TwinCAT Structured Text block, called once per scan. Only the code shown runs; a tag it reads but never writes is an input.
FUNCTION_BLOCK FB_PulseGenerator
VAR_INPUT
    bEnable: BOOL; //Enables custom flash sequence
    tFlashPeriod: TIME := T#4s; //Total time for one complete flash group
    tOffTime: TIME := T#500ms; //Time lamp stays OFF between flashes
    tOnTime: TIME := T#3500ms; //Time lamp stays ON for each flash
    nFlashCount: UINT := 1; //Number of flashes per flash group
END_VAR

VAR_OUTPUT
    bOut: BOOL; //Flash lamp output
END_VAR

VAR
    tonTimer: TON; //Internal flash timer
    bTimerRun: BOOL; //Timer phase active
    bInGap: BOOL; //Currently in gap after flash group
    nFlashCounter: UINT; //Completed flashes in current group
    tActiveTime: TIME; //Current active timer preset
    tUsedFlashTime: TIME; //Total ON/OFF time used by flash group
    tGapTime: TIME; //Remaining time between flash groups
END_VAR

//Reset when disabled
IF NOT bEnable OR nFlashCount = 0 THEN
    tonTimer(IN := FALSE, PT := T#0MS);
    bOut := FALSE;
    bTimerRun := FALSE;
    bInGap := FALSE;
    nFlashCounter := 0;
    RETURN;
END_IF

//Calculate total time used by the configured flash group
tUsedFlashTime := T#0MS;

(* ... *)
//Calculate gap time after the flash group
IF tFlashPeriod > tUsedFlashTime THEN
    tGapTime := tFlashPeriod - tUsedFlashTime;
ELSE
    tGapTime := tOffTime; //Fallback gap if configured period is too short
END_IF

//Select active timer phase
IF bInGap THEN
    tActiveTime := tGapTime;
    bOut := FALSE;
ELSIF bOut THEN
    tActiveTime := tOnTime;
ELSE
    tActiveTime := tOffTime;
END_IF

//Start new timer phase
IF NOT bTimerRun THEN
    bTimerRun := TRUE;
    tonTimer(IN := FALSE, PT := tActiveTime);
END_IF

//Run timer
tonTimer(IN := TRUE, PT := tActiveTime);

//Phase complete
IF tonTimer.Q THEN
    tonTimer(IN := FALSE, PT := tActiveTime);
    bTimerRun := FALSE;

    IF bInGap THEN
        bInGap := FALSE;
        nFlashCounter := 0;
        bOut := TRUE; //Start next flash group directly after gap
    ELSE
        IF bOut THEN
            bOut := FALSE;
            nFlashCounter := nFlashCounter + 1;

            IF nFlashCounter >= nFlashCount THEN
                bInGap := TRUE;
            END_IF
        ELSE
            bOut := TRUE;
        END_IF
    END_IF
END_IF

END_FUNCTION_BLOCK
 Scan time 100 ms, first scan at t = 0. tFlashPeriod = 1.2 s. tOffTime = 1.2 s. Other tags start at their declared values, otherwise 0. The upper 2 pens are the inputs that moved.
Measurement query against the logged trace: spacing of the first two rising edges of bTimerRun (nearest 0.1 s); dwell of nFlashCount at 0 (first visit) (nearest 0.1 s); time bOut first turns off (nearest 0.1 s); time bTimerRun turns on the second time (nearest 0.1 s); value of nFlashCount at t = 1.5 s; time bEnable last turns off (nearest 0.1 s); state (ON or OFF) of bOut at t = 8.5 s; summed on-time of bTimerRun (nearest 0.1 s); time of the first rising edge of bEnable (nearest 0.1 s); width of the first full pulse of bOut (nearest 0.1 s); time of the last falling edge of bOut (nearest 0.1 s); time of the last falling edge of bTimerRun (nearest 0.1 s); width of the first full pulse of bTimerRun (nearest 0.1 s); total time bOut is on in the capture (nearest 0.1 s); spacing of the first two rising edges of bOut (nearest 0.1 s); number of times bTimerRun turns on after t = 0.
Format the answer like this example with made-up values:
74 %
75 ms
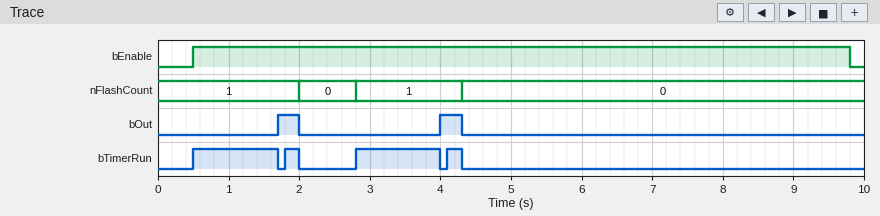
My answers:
1.3 s
0.8 s
2.0 s
1.8 s
1
9.8 s
OFF
2.8 s
0.5 s
0.3 s
4.3 s
4.3 s
1.2 s
0.6 s
2.3 s
4
